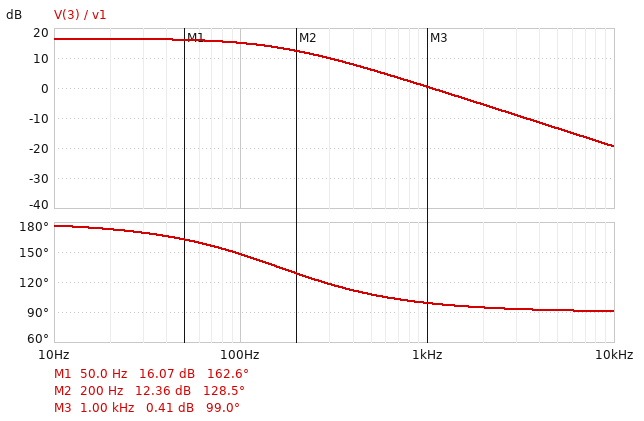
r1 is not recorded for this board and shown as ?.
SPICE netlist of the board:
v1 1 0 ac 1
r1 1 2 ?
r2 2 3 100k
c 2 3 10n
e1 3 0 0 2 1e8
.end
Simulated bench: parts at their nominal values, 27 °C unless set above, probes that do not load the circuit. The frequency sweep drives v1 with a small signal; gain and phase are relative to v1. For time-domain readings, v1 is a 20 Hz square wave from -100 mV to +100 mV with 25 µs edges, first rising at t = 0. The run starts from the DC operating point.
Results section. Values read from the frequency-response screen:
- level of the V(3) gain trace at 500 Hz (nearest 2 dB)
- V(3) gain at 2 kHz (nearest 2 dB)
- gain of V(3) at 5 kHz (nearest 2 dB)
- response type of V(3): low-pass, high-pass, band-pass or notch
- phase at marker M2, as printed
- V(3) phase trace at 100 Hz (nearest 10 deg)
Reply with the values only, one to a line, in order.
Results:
6 dB
-6 dB
-14 dB
low-pass
128.5 deg
150 deg
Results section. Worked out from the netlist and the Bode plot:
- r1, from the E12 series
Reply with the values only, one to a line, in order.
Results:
15 kΩ
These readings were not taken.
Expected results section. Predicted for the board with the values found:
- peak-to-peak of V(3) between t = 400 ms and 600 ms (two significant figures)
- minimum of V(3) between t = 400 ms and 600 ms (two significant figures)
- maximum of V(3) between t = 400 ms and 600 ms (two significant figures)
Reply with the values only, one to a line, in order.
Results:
1.3 V
-670 mV
670 mV
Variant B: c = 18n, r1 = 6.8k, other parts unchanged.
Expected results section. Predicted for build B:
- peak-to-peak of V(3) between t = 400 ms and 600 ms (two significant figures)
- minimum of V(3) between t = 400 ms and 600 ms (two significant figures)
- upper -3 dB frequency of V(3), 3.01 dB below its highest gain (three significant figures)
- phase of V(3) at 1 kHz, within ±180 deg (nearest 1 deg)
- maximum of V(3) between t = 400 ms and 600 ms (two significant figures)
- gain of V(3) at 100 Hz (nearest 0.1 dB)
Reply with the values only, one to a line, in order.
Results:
2.9 V
-1.5 V
88.4 Hz
95 deg
1.5 V
19.8 dB
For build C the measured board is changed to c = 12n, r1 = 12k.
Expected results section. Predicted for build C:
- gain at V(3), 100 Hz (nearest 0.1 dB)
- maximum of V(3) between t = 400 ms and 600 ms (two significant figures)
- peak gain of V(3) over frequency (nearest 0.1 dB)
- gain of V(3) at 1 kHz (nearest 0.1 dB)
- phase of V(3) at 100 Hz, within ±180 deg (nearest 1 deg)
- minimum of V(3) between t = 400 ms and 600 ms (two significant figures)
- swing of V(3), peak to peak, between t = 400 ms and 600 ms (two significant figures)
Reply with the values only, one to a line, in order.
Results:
16.5 dB
830 mV
18.4 dB
0.8 dB
143 deg
-830 mV
1.7 V
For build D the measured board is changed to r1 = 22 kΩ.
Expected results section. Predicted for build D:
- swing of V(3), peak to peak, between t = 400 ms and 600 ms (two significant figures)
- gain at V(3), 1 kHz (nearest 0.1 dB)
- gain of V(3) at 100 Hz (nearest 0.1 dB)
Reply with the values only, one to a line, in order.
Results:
910 mV
-2.9 dB
11.7 dB
